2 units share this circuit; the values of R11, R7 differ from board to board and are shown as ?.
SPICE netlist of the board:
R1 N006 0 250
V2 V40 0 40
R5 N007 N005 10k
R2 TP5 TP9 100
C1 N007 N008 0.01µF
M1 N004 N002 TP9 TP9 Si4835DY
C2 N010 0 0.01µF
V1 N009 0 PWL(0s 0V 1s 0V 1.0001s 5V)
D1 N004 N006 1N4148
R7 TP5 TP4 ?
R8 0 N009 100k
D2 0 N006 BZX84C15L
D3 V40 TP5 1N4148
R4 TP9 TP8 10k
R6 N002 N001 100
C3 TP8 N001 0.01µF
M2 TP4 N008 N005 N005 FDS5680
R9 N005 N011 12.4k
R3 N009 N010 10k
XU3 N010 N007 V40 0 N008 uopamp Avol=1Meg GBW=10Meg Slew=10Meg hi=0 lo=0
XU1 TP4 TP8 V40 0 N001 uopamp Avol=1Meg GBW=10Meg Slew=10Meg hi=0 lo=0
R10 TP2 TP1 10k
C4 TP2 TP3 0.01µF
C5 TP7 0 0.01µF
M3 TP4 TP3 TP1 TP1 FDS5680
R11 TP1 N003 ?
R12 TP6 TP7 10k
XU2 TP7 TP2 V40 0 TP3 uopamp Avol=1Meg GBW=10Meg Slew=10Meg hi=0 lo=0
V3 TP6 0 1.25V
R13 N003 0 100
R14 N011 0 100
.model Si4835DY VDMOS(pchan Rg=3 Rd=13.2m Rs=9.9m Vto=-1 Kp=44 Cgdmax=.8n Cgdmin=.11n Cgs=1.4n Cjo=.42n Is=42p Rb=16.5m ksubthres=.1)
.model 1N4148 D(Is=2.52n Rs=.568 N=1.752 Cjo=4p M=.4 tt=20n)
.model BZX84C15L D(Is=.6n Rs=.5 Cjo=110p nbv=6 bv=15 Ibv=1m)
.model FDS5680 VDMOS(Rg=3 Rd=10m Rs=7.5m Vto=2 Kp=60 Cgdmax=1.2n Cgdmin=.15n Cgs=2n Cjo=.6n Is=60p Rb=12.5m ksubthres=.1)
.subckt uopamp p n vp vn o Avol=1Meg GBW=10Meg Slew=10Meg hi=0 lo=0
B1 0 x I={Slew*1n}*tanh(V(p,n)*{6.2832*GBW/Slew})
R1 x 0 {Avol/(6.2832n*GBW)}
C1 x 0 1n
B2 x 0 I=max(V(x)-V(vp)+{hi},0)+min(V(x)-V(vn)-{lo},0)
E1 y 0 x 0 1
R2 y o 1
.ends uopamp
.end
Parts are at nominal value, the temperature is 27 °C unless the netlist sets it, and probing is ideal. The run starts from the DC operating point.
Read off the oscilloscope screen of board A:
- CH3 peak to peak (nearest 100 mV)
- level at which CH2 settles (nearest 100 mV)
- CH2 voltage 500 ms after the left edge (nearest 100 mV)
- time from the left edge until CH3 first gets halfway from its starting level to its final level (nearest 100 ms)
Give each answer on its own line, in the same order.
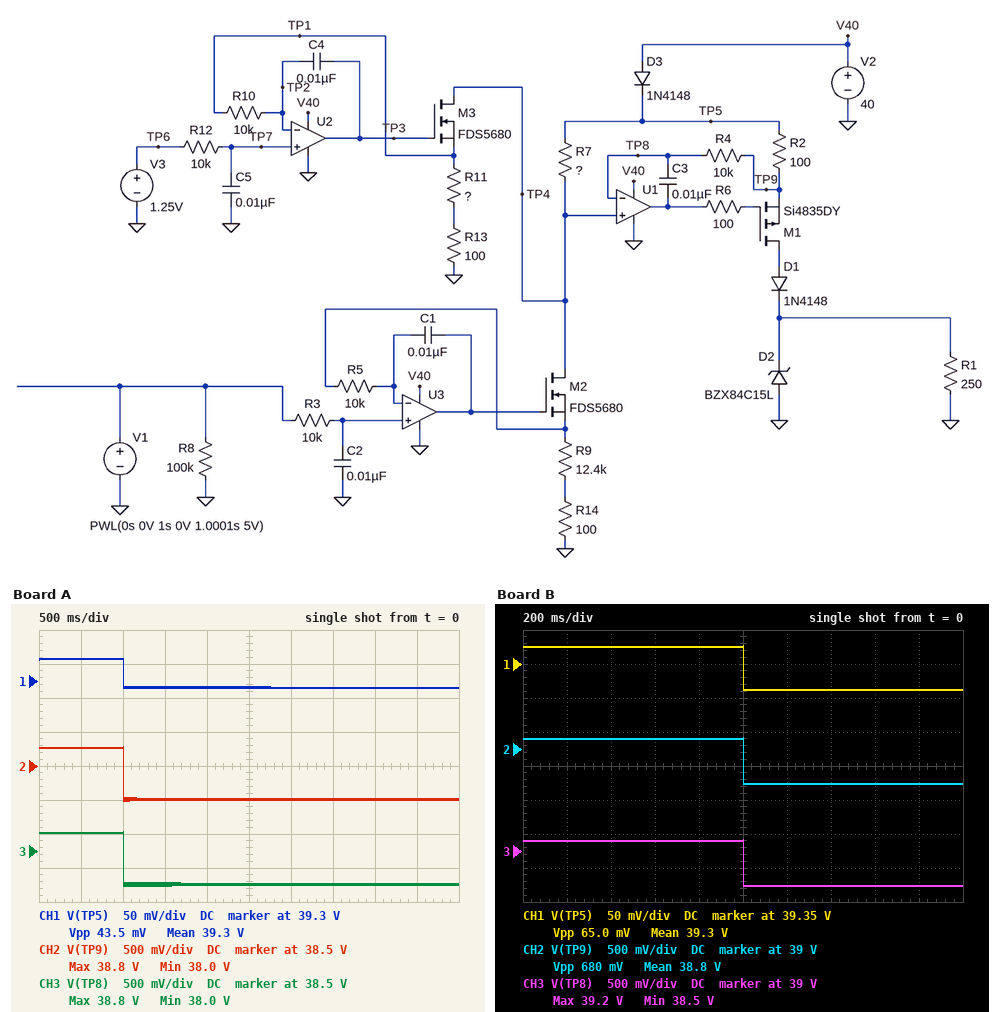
800 mV
38.0 V
38.8 V
1.0 s
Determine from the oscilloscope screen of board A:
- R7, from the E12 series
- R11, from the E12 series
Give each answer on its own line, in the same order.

1.8 kΩ
3.9 kΩ
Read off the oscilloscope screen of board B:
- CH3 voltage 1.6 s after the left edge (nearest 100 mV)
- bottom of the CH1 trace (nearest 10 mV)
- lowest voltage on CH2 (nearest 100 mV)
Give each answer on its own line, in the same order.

38.5 V
39.31 V
38.5 V
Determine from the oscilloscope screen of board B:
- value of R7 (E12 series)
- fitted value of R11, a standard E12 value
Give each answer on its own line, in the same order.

1.5 kΩ
8.2 kΩ
